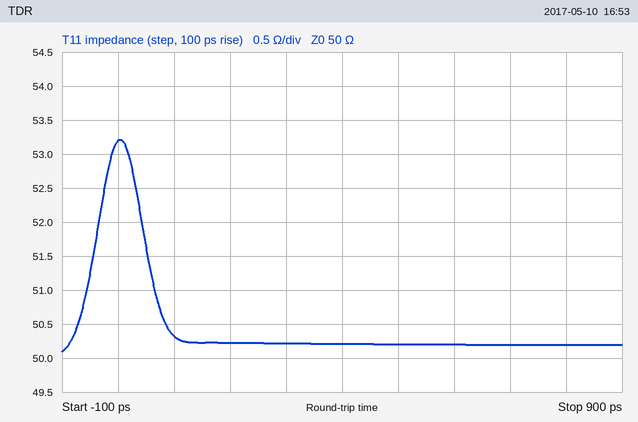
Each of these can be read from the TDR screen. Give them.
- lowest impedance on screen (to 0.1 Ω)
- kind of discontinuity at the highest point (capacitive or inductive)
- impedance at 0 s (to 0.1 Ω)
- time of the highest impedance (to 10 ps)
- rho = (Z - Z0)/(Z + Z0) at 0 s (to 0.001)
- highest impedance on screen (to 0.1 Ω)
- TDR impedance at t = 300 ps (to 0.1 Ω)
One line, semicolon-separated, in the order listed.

50.1 Ω; inductive; 53.2 Ω; 0 ps; +0.031; 53.2 Ω; 50.2 Ω
